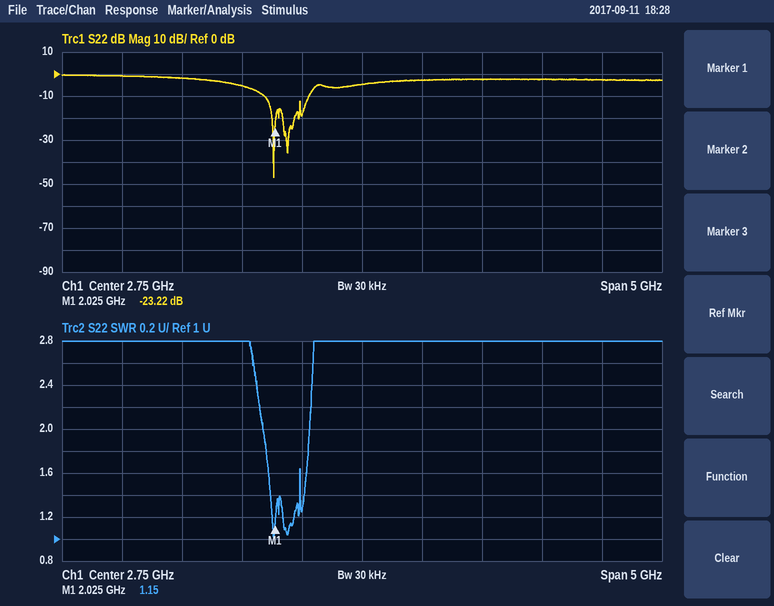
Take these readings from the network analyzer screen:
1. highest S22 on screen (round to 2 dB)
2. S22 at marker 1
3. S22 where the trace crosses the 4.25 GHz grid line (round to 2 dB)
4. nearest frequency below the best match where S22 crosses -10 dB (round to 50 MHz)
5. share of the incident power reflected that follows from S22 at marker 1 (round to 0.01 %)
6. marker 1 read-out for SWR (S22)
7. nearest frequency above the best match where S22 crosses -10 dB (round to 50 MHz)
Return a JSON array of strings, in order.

["0 dB", "-23.22 dB", "-2 dB", "1.95 GHz", "0.48 %", "1.15", "2.30 GHz"]
